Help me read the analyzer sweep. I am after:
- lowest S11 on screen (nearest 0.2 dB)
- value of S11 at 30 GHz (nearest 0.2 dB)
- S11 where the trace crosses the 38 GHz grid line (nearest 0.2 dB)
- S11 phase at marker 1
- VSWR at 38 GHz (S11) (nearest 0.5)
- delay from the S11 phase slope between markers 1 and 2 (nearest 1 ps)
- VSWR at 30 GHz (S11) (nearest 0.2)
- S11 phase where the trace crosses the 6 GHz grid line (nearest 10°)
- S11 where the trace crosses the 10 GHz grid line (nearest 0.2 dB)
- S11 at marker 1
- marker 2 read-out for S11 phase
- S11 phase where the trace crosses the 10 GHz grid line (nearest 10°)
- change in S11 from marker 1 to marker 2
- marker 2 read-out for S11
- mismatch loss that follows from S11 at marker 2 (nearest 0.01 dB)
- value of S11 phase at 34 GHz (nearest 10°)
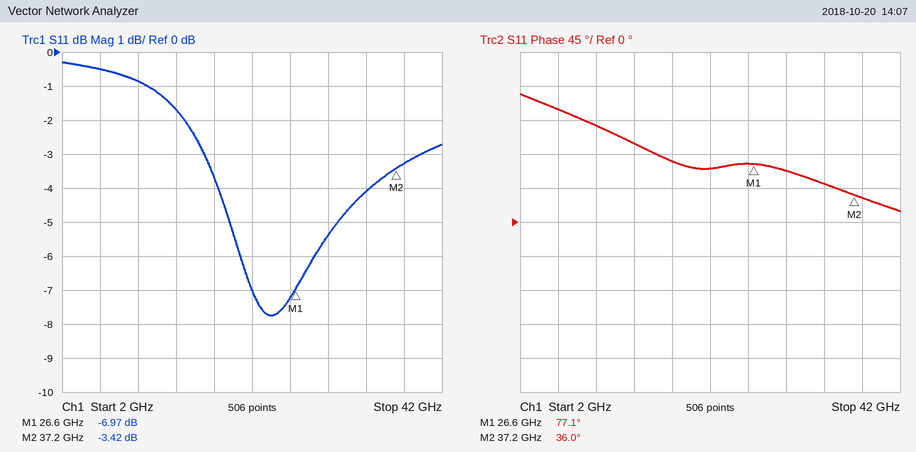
-7.8 dB
-5.4 dB
-3.2 dB
77.1°
5.5
11 ps
3.4
150°
-0.8 dB
-6.97 dB
36.0°
130°
3.55 dB
-3.42 dB
2.64 dB
50°
